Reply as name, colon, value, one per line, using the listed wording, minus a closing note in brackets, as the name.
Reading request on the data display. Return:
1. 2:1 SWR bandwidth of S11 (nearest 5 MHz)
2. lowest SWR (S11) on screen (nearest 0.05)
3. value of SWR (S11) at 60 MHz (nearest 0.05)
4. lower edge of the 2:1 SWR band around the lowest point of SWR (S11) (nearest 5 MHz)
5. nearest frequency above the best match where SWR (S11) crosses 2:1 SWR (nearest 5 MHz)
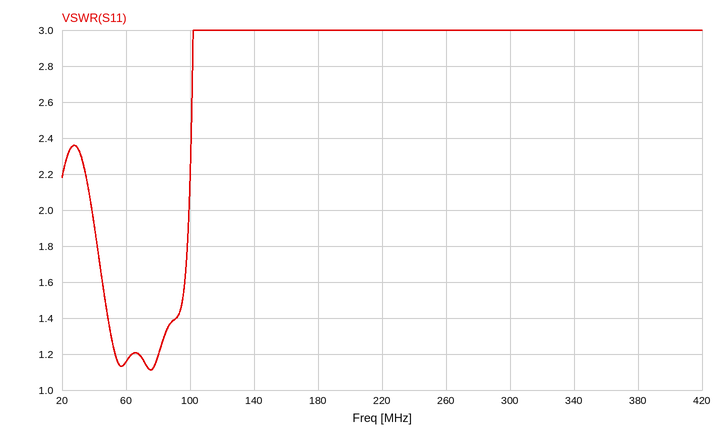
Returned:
2:1 SWR bandwidth of S11: 60 MHz
lowest SWR (S11) on screen: 1.10
value of SWR (S11) at 60 MHz: 1.15
lower edge of the 2:1 SWR band around the lowest point of SWR (S11): 40 MHz
nearest frequency above the best match where SWR (S11) crosses 2:1 SWR: 100 MHz
